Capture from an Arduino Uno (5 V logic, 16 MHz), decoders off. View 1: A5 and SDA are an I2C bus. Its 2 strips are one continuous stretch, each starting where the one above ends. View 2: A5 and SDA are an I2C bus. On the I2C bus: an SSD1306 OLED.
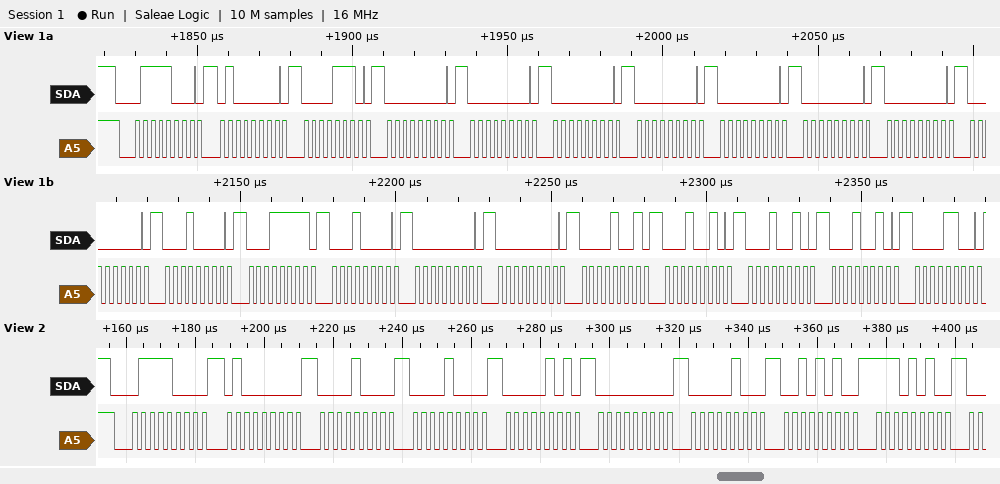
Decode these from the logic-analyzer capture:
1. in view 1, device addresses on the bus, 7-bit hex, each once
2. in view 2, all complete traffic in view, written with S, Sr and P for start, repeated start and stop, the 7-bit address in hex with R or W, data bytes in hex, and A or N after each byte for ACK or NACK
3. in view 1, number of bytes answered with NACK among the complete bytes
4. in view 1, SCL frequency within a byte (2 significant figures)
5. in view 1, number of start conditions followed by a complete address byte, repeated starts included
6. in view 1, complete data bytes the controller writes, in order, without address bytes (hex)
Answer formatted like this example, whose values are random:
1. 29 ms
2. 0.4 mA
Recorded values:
1. 0x3C
2. S 3CW A 40 A 08 A 08 A 05 A 00 A 04 A 2A A EA A
3. 0
4. 400 kHz
5. 1
6. 40 0E 00 00 00 00 00 00 00 00 10 1F 10 00 00 09 12 12 12 0C
